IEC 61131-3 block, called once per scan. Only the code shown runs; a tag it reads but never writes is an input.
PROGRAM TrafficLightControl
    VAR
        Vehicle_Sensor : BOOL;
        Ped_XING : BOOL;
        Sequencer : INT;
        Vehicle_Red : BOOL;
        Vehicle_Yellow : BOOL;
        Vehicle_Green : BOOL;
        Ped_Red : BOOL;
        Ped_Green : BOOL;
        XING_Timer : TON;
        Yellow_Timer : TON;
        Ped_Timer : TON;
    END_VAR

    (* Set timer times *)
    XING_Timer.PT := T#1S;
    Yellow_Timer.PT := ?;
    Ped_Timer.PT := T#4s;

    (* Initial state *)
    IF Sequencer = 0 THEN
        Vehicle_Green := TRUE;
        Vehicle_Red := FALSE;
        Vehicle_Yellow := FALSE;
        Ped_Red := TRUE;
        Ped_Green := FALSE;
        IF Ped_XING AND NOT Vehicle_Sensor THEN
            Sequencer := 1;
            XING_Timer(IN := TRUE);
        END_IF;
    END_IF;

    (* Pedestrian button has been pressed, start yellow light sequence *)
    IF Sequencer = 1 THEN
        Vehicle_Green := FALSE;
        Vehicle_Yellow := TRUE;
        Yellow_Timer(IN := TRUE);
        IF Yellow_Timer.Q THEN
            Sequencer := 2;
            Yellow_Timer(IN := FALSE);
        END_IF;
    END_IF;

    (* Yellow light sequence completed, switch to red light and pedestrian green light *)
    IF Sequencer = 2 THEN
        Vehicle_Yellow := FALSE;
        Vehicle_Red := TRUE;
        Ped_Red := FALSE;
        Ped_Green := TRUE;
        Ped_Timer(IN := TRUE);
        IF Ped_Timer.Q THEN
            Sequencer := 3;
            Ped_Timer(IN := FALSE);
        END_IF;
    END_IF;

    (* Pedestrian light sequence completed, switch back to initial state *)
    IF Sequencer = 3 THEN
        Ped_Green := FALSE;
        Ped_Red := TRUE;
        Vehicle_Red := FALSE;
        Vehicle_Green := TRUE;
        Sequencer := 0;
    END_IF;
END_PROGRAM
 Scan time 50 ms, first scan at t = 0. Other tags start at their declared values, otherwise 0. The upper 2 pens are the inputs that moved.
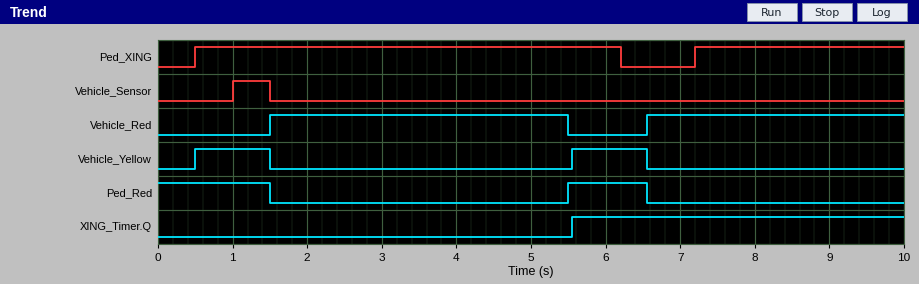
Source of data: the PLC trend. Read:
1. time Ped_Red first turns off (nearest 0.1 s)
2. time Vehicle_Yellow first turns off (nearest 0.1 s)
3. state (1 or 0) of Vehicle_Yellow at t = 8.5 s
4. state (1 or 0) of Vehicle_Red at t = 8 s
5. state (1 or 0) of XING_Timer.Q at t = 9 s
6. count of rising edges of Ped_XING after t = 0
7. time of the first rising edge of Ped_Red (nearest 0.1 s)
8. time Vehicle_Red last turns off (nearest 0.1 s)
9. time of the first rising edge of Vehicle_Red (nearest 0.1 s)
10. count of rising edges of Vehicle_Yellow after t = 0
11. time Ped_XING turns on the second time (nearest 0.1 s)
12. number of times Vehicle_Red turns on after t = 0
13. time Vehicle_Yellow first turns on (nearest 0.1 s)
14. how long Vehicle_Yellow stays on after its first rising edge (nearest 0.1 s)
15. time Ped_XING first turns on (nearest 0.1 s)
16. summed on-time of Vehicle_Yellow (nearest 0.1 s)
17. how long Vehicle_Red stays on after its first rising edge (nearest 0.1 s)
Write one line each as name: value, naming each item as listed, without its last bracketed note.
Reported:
time Ped_Red first turns off: 1.5 s
time Vehicle_Yellow first turns off: 1.5 s
state (1 or 0) of Vehicle_Yellow at t = 8.5 s: 0
state (1 or 0) of Vehicle_Red at t = 8 s: 1
state (1 or 0) of XING_Timer.Q at t = 9 s: 1
count of rising edges of Ped_XING after t = 0: 2
time of the first rising edge of Ped_Red: 5.5 s
time Vehicle_Red last turns off: 5.5 s
time of the first rising edge of Vehicle_Red: 1.5 s
count of rising edges of Vehicle_Yellow after t = 0: 2
time Ped_XING turns on the second time: 7.2 s
number of times Vehicle_Red turns on after t = 0: 2
time Vehicle_Yellow first turns on: 0.5 s
how long Vehicle_Yellow stays on after its first rising edge: 1.0 s
time Ped_XING first turns on: 0.5 s
summed on-time of Vehicle_Yellow: 2.0 s
how long Vehicle_Red stays on after its first rising edge: 4.0 s
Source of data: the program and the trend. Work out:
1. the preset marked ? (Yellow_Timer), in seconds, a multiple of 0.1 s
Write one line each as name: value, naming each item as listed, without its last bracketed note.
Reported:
the preset marked ? (Yellow_Timer), in seconds, a multiple of 0.1 s: 1.0 s
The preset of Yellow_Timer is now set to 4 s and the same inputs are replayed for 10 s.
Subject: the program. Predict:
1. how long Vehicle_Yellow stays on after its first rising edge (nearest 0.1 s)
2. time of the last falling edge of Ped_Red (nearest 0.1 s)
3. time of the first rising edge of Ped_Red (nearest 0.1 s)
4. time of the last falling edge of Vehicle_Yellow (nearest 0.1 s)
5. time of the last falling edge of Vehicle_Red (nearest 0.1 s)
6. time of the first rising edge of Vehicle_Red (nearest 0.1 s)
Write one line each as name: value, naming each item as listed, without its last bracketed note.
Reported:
how long Vehicle_Yellow stays on after its first rising edge: 4.0 s
time of the last falling edge of Ped_Red: 4.5 s
time of the first rising edge of Ped_Red: 8.5 s
time of the last falling edge of Vehicle_Yellow: 4.5 s
time of the last falling edge of Vehicle_Red: 8.5 s
time of the first rising edge of Vehicle_Red: 4.5 s
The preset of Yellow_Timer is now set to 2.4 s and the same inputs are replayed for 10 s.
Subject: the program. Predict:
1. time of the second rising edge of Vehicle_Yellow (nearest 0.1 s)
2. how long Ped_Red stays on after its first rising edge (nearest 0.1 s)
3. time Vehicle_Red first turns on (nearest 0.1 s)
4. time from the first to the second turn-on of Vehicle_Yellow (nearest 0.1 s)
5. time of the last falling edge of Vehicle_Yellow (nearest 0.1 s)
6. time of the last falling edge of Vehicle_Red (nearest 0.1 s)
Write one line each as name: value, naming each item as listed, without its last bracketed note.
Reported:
time of the second rising edge of Vehicle_Yellow: 7.2 s
how long Ped_Red stays on after its first rising edge: 2.7 s
time Vehicle_Red first turns on: 2.9 s
time from the first to the second turn-on of Vehicle_Yellow: 6.7 s
time of the last falling edge of Vehicle_Yellow: 9.6 s
time of the last falling edge of Vehicle_Red: 6.9 s
